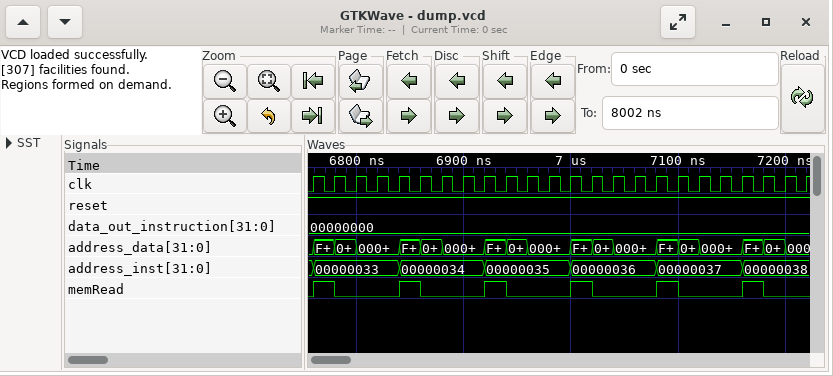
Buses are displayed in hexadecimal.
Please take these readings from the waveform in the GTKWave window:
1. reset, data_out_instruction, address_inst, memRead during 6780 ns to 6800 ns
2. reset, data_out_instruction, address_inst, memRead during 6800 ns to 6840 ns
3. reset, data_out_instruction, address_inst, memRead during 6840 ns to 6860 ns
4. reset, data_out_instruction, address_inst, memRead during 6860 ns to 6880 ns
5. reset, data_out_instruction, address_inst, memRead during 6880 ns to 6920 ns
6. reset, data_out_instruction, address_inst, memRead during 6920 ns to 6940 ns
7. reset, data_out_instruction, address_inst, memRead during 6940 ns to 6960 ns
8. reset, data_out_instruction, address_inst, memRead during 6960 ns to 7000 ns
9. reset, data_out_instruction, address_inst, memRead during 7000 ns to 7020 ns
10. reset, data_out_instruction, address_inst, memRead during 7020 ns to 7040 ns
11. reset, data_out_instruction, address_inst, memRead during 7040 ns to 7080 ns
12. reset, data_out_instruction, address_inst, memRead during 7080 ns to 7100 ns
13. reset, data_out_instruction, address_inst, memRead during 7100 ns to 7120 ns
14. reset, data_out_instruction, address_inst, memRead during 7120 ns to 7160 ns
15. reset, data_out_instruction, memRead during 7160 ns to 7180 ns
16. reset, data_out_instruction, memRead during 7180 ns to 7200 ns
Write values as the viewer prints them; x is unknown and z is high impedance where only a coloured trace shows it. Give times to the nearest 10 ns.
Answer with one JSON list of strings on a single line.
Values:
["reset=1, data_out_instruction=00000000, address_inst=00000033, memRead=0", "reset=1, data_out_instruction=00000000, address_inst=00000033, memRead=0", "reset=1, data_out_instruction=00000000, address_inst=00000034, memRead=1", "reset=1, data_out_instruction=00000000, address_inst=00000034, memRead=0", "reset=1, data_out_instruction=00000000, address_inst=00000034, memRead=0", "reset=1, data_out_instruction=00000000, address_inst=00000035, memRead=1", "reset=1, data_out_instruction=00000000, address_inst=00000035, memRead=0", "reset=1, data_out_instruction=00000000, address_inst=00000035, memRead=0", "reset=1, data_out_instruction=00000000, address_inst=00000036, memRead=1", "reset=1, data_out_instruction=00000000, address_inst=00000036, memRead=0", "reset=1, data_out_instruction=00000000, address_inst=00000036, memRead=0", "reset=1, data_out_instruction=00000000, address_inst=00000037, memRead=1", "reset=1, data_out_instruction=00000000, address_inst=00000037, memRead=0", "reset=1, data_out_instruction=00000000, address_inst=00000037, memRead=0", "reset=1, data_out_instruction=00000000, memRead=1", "reset=1, data_out_instruction=00000000, memRead=0"]
